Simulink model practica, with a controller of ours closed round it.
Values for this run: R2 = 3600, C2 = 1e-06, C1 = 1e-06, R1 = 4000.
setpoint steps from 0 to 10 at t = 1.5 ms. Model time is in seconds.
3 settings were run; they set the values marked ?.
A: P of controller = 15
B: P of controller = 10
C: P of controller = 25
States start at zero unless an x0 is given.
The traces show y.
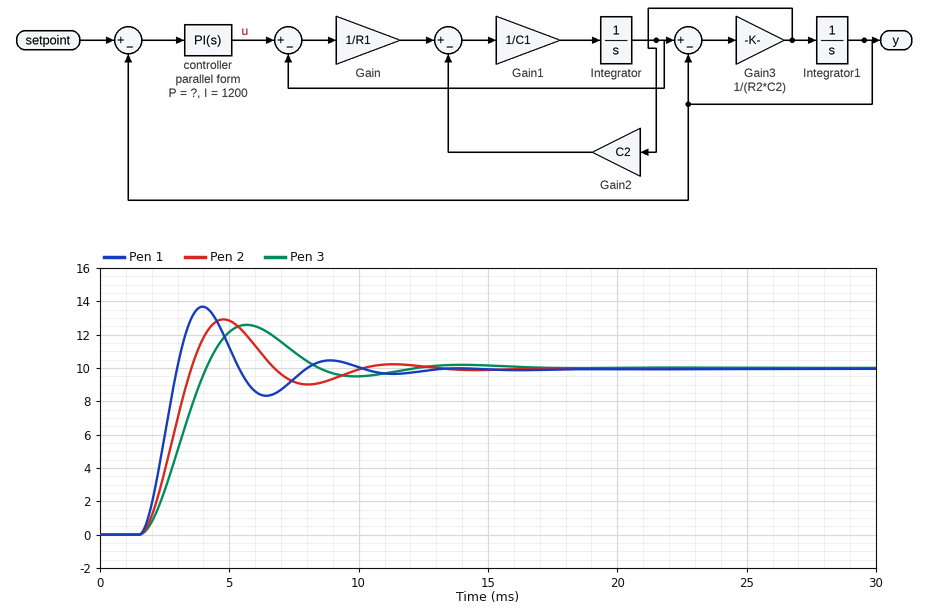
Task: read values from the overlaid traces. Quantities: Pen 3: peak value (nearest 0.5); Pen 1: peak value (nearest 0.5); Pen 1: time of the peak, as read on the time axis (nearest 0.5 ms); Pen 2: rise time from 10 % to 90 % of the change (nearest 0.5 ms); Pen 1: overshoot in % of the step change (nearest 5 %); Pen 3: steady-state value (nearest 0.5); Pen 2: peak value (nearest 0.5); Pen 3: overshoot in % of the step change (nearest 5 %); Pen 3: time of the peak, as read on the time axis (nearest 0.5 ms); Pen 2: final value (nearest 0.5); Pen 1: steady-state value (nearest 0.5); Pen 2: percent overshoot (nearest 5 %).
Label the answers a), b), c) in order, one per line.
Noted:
a) 12.5
b) 13.5
c) 4.0 ms
d) 1.5 ms
e) 35 %
f) 10.0
g) 13.0
h) 25 %
i) 5.5 ms
j) 10.0
k) 10.0
l) 30 %
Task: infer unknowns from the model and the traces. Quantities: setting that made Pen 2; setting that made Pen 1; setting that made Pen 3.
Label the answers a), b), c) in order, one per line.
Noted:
a) A
b) C
c) B
